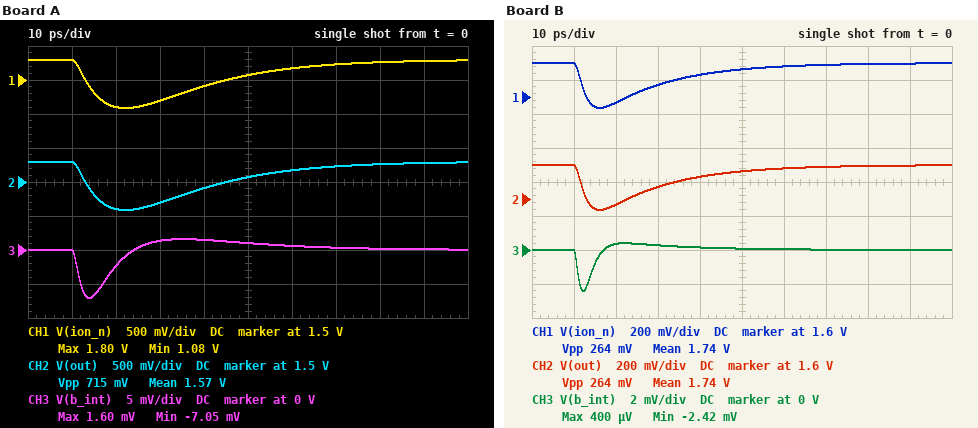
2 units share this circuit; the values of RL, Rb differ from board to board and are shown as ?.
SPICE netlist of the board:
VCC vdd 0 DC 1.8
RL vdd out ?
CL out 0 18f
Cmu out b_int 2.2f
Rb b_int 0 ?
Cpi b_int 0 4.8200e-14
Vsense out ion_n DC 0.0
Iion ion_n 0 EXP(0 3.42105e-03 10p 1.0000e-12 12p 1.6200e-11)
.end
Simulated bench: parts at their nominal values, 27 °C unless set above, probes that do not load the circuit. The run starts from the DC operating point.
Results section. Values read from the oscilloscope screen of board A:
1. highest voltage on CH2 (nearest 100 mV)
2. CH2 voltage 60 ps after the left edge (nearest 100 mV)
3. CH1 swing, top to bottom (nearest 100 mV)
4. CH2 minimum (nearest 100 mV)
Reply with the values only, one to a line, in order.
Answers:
1.8 V
1.7 V
700 mV
1.1 V
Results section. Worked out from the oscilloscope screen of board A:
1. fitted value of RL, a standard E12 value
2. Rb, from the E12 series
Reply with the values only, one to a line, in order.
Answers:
390 Ω
33 Ω
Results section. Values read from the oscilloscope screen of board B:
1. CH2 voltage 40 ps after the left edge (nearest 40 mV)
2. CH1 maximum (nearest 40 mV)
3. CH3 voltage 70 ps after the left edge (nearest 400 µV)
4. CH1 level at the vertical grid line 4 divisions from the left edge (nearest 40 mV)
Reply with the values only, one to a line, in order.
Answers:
1.72 V
1.80 V
0 V
1.72 V
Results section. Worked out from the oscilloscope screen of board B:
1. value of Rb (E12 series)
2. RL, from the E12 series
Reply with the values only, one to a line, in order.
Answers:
15 Ω
100 Ω
